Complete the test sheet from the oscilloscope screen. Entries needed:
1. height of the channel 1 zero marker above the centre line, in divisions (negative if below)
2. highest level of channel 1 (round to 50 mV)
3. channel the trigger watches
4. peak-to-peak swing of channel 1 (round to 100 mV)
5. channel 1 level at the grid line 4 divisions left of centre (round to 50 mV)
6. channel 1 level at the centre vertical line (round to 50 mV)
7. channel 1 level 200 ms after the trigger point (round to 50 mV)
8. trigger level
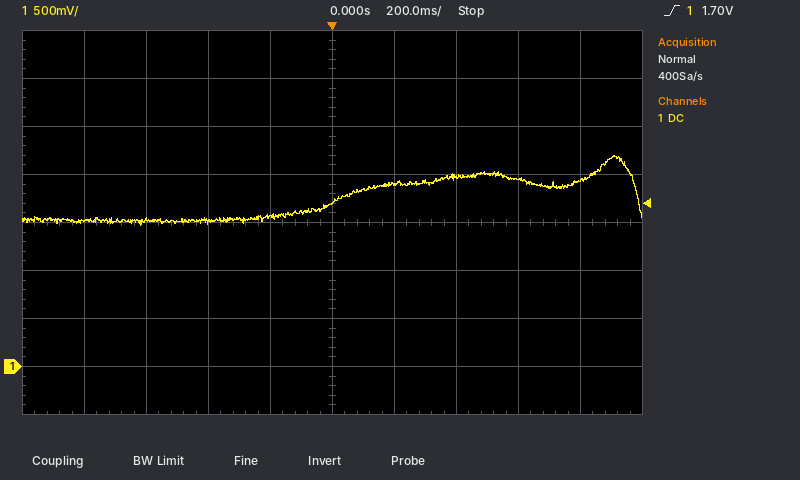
-3.0 div
2.20 V
channel 1
700 mV
1.50 V
1.70 V
1.90 V
1.70 V
